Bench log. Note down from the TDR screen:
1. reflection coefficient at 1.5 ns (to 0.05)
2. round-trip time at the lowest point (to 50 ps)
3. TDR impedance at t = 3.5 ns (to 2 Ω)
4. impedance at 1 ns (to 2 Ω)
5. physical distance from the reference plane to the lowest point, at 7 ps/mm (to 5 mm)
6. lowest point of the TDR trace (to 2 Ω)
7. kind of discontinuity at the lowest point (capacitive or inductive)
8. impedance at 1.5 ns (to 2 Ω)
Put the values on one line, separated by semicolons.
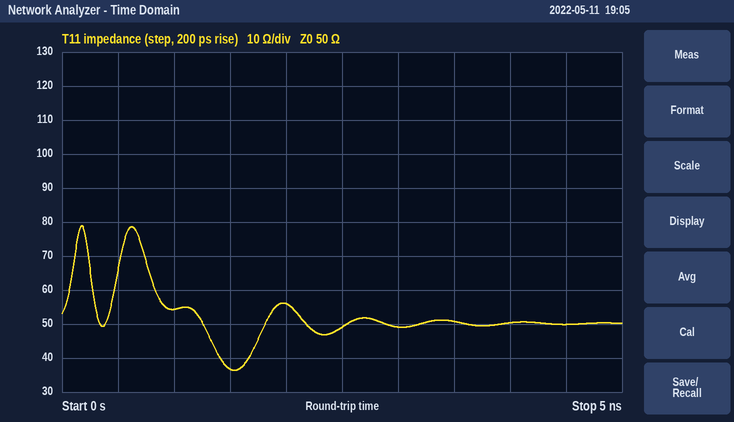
-0.15; 1.55 ns; 50 Ω; 54 Ω; 110 mm; 36 Ω; capacitive; 36 Ω
